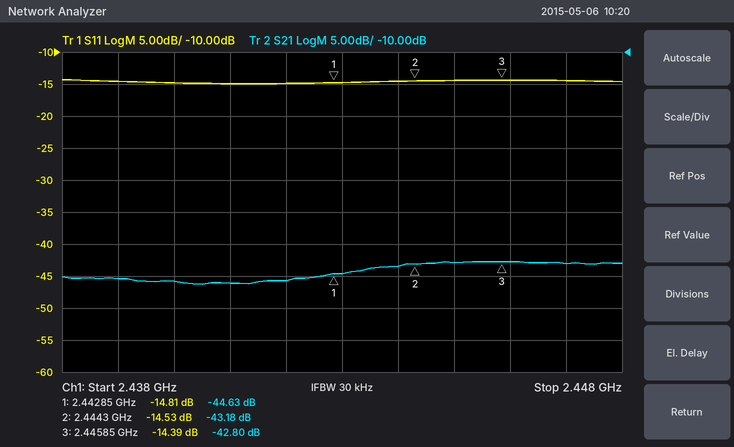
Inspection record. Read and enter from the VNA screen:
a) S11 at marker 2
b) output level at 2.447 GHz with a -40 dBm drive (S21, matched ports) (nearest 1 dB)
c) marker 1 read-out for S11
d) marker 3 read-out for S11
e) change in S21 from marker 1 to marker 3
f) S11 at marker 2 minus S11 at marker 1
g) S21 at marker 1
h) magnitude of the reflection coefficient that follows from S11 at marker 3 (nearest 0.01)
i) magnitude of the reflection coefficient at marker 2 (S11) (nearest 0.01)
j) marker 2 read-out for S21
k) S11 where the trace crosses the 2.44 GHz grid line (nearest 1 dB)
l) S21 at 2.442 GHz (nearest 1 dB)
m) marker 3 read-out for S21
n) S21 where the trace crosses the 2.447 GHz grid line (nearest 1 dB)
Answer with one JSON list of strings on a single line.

["-14.53 dB", "-83 dBm", "-14.81 dB", "-14.39 dB", "1.83 dB", "0.28 dB", "-44.63 dB", "0.19", "0.19", "-43.18 dB", "-15 dB", "-46 dB", "-42.80 dB", "-43 dB"]
